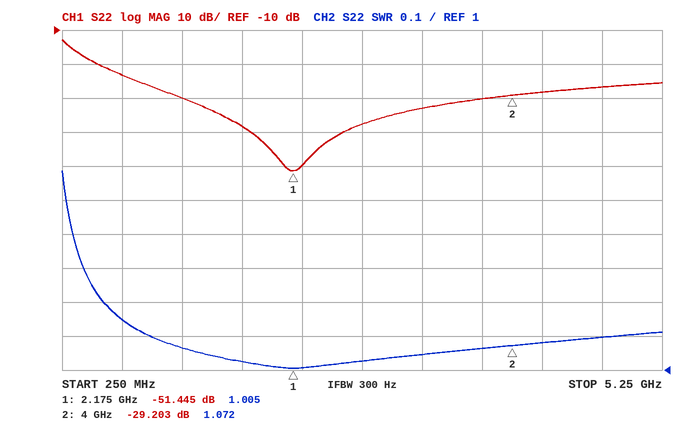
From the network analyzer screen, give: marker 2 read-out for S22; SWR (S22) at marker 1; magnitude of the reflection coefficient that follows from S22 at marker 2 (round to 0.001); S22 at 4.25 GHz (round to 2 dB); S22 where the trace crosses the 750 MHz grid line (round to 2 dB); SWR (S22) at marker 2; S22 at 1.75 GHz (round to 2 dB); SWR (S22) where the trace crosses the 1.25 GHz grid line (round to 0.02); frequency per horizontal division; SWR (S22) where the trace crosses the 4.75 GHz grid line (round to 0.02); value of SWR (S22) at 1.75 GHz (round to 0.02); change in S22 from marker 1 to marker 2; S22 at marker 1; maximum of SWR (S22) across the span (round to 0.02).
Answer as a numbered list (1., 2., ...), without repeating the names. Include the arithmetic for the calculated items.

1. -29.203 dB
2. 1.005
3. 10^(-29.203/20) ≈ 0.035
4. -28 dB
5. -24 dB
6. 1.072
7. -38 dB
8. 1.06
9. 500 MHz
10. 1.10
11. 1.02
12. -29.203 − (-51.445) = 22.242 dB
13. -51.445 dB
14. 1.58
